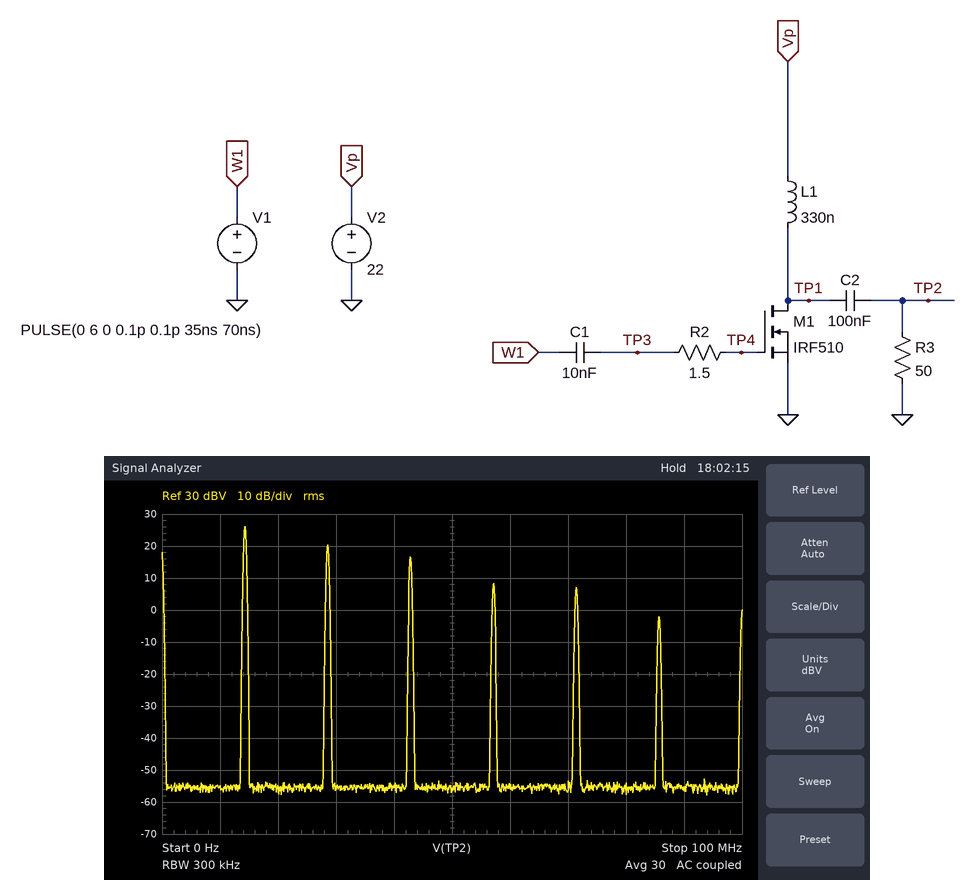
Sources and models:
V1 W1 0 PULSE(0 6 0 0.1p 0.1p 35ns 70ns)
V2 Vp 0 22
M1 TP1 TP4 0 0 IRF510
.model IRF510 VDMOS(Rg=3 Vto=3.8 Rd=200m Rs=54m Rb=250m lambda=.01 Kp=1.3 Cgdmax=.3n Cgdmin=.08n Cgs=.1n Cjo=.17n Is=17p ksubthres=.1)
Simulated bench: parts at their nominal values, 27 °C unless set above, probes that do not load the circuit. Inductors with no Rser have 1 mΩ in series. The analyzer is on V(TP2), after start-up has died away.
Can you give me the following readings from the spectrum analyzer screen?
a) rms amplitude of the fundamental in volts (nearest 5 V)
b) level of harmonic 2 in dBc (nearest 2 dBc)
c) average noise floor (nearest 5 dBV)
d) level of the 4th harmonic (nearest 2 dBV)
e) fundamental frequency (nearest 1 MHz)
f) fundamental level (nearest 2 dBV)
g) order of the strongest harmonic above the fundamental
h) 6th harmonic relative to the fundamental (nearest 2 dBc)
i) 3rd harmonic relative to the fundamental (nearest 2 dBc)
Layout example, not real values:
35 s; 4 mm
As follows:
20 V; -6 dBc; -55 dBV; 8 dBV; 14 MHz; 26 dBV; 2; -28 dBc; -10 dBc
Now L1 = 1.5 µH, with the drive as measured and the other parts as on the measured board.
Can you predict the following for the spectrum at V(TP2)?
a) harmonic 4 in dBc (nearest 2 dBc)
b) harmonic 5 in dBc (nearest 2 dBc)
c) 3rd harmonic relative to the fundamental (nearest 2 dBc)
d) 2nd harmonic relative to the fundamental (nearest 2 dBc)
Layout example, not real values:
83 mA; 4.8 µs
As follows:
-32 dBc; -24 dBc; -14 dBc; -20 dBc
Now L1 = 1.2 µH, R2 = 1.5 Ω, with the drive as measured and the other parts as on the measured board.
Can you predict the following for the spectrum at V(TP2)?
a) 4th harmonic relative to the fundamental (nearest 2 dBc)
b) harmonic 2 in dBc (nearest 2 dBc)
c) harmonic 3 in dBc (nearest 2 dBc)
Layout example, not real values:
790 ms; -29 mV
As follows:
-30 dBc; -18 dBc; -14 dBc
